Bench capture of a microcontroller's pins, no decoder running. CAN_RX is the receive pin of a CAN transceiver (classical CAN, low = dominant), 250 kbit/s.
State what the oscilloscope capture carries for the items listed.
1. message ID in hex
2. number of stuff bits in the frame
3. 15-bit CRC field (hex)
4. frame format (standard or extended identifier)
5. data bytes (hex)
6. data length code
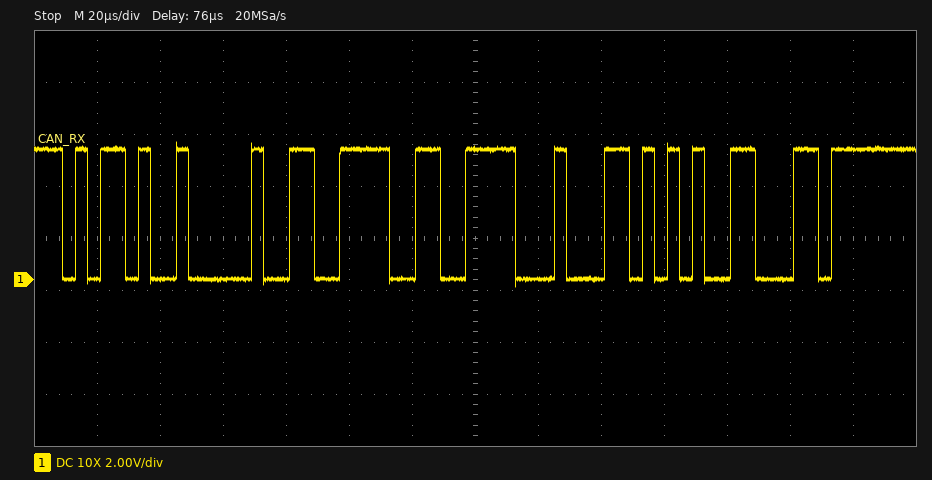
0x5A4
1
0x5531
standard
3C CF 11
3
